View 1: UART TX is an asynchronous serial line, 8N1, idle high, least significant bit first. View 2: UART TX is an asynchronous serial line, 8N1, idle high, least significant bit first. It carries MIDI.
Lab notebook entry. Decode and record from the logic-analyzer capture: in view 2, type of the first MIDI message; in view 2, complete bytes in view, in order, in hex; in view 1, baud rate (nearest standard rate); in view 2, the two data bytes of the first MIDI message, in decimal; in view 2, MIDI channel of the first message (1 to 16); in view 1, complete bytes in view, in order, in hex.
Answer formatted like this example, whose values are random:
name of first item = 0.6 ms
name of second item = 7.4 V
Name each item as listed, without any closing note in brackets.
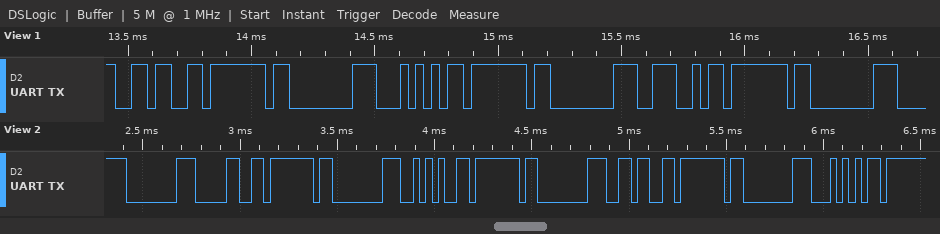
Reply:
in view 2, type of the first MIDI message = Note Off
in view 2, complete bytes in view, in order, in hex = 0x80 0x30 0x7F 0x80 0x2A 0x7F 0x80 0x36 0x7F 0x80 0x54
in view 1, baud rate = 31250 baud
in view 2, the two data bytes of the first MIDI message, in decimal = 48, 127
in view 2, MIDI channel of the first message = 1
in view 1, complete bytes in view, in order, in hex = 0x36 0x7F 0x80 0x54 0x7F 0x80 0x4E 0x7F 0x80
